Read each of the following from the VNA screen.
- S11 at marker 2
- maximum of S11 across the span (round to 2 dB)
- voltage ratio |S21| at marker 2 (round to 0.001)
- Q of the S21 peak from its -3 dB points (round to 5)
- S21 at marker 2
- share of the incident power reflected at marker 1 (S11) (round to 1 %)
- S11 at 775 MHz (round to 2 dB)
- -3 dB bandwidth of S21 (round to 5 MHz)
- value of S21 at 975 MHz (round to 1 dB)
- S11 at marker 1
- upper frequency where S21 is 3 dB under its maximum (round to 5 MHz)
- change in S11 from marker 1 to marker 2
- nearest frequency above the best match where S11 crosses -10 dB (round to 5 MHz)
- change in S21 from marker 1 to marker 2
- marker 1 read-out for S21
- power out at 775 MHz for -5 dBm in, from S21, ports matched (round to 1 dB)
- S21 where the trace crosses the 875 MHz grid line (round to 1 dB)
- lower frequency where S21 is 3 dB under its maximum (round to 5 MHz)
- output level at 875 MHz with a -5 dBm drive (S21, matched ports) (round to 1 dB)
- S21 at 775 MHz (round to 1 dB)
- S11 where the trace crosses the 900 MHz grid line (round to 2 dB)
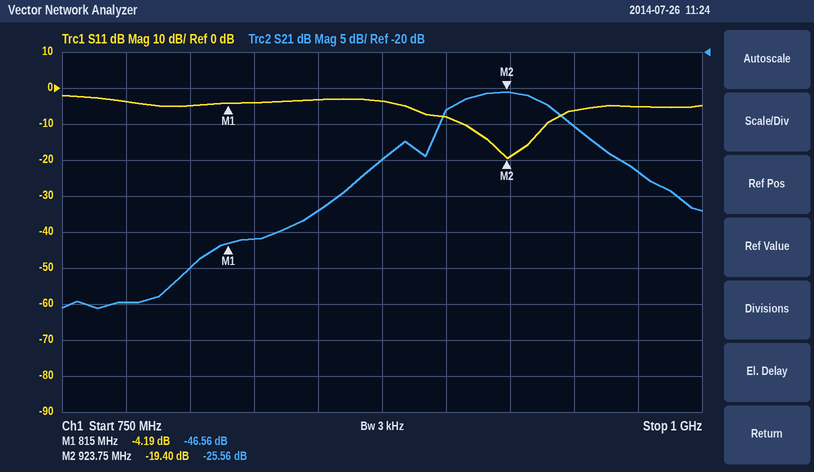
-19.40 dB
-2 dB
0.053
20
-25.56 dB
38 %
-4 dB
45 MHz
-37 dB
-4.19 dB
945 MHz
-15.21 dB
940 MHz
21.00 dB
-46.56 dB
-60 dBm
-35 dB
900 MHz
-40 dBm
-55 dB
-8 dB
